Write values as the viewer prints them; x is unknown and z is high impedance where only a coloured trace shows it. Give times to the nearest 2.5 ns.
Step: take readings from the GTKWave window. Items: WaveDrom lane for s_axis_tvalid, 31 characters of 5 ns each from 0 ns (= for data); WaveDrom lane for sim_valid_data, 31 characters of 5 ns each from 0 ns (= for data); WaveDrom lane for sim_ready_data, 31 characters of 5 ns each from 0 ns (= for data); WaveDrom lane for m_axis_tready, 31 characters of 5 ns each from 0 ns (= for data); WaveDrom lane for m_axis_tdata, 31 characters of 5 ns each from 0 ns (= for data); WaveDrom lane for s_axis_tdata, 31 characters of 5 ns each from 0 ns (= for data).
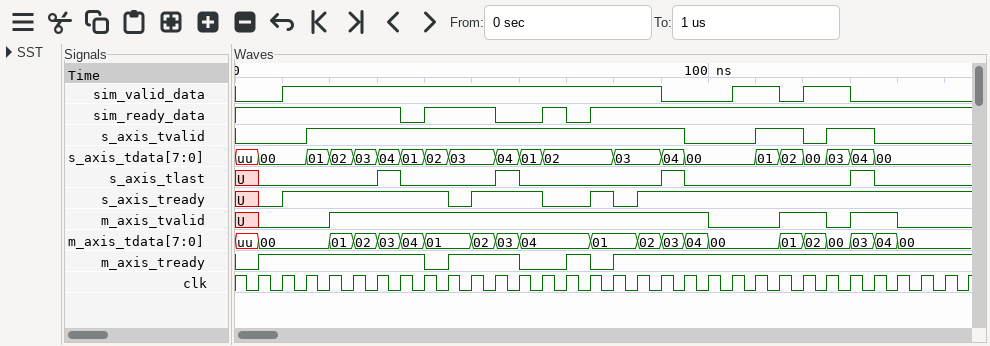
{name: 's_axis_tvalid', wave: '0..1...............0..1.01.0...'}
{name: 'sim_valid_data', wave: '0.1...............0..1.01.0....'}
{name: 'sim_ready_data', wave: '1......01..0.101...............'}
{name: 'm_axis_tready', wave: '01......01..0.101..............'}
{name: 'm_axis_tdata', wave: 'x=..=====.===..=.====..======..', data: '00 01 02 03 04 01 02 03 04 01 02 03 04 00 01 02 00 03 04 00'}
{name: 's_axis_tdata', wave: 'x=.=======.===..=.==..======...', data: '00 01 02 03 04 01 02 03 04 01 02 03 04 00 01 02 00 03 04 00'}
